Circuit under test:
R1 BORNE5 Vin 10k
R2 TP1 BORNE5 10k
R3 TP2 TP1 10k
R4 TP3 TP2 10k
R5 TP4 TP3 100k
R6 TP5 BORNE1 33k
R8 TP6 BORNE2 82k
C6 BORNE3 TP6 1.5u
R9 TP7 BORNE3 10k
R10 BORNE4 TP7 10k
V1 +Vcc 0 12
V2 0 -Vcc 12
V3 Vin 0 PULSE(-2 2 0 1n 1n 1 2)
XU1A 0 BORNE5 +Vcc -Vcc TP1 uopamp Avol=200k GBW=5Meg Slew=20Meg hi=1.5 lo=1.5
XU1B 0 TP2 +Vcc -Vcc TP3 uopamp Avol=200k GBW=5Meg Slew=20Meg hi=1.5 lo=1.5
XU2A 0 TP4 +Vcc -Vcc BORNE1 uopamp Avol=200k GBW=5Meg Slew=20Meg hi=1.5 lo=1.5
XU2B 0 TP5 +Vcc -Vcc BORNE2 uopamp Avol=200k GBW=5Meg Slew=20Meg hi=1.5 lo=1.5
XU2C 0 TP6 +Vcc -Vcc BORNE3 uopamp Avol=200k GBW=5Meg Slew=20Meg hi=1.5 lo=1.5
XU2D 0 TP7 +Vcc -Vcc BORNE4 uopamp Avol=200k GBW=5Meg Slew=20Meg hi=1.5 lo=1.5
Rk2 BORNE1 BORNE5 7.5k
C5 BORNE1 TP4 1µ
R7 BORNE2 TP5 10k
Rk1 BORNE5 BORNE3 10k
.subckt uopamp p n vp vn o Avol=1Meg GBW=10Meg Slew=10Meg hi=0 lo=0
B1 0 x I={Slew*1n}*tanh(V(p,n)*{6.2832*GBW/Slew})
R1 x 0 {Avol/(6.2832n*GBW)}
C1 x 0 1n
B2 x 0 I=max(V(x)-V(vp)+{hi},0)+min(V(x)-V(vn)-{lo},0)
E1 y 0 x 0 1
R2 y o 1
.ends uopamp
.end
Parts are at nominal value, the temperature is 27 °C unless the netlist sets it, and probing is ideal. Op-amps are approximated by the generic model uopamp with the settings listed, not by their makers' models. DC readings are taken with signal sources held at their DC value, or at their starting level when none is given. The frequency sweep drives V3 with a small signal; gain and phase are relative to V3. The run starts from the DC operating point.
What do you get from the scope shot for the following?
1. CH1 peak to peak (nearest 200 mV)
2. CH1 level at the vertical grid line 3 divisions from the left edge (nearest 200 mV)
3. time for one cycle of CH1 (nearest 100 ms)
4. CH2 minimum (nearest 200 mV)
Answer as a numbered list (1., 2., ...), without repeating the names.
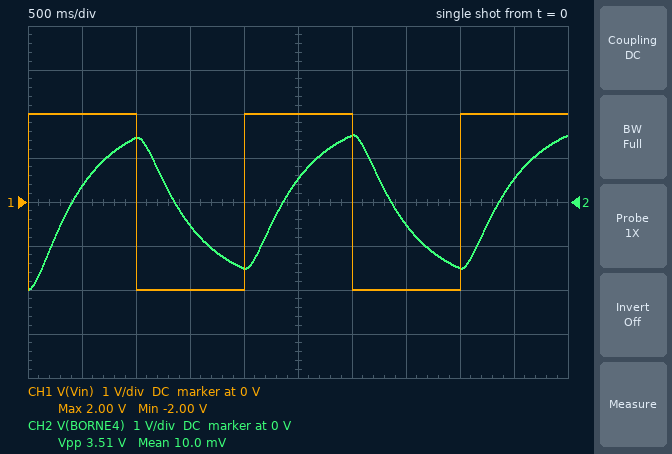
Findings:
1. 4.0 V
2. -2.0 V
3. 2.0 s
4. -2.0 V
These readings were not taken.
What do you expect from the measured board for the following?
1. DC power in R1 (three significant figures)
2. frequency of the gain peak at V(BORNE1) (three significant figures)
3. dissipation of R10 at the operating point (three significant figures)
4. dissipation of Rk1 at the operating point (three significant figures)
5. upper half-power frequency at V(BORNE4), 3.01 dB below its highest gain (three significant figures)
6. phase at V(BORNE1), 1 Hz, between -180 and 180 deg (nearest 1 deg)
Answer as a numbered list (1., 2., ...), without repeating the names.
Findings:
1. 400 µW
2. 790 mHz
3. 400 µW
4. 400 µW
5. 340 mHz
6. 170 deg
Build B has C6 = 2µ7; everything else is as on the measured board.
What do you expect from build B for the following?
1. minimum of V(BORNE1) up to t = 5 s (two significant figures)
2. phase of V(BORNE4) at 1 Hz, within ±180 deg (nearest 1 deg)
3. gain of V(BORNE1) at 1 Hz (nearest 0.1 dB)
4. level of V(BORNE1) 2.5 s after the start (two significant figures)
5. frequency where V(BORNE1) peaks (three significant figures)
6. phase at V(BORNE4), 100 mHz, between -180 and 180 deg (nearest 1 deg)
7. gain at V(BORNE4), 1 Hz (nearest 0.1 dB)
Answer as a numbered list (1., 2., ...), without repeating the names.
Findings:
1. -2.6 V
2. -107 deg
3. -2.9 dB
4. -1.6 V
5. 589 mHz
6. -32 deg
7. -16.1 dB
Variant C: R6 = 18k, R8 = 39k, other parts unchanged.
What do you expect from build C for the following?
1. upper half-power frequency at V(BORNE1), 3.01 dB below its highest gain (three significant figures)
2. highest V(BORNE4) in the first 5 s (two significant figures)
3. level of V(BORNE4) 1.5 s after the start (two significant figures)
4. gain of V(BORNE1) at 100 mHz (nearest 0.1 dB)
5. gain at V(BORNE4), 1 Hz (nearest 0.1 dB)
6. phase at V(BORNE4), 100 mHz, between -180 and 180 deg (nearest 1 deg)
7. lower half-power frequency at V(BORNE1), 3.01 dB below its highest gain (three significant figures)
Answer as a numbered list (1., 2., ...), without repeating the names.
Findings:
1. 2.94 Hz
2. 2.2 V
3. -2.2 V
4. -23.6 dB
5. -0.5 dB
6. -5 deg
7. 818 mHz
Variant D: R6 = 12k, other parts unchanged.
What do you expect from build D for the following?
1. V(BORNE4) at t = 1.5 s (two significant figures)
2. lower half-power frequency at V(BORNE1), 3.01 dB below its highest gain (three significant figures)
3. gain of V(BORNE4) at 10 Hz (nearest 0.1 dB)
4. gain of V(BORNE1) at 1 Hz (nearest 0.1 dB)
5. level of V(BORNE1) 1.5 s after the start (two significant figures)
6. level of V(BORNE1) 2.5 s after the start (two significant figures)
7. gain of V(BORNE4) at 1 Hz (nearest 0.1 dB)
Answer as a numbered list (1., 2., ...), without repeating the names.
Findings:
1. -2.0 V
2. 625 mHz
3. -35.4 dB
4. -3.0 dB
5. 200 mV
6. -200 mV
7. -2.3 dB
